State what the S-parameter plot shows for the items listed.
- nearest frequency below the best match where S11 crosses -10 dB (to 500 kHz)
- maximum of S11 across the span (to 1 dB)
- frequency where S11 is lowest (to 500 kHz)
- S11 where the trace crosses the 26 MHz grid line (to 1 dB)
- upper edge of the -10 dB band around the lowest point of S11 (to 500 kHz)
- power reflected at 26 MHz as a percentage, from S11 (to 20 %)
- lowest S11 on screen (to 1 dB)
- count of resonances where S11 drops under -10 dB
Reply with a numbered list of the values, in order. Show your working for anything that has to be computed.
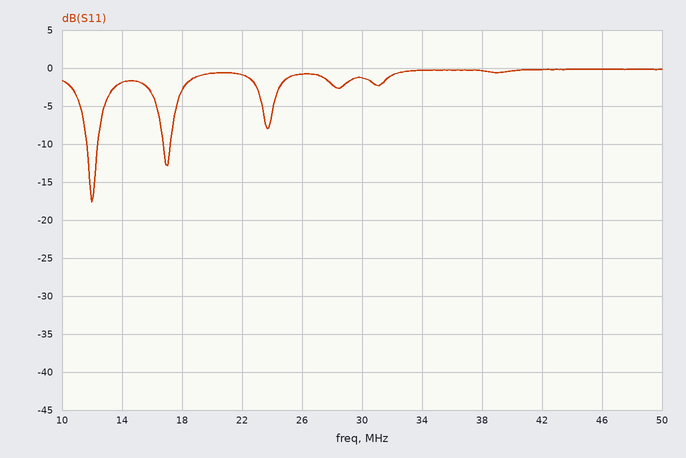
1. 11.5 MHz
2. 0 dB
3. 12.0 MHz
4. -1 dB
5. 12.5 MHz
6. 10^(-1/10) ≈ 79.4 %, so 80 % to the nearest 20 %
7. -18 dB
8. 2
